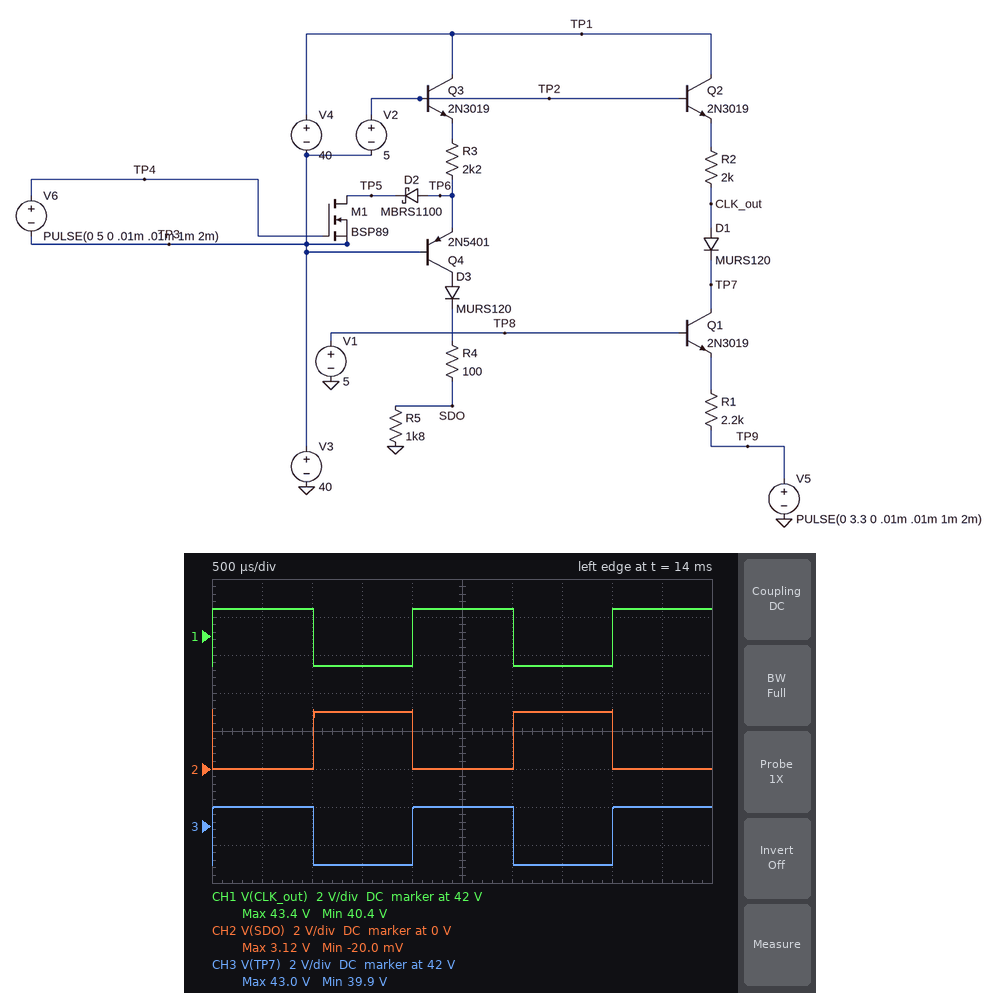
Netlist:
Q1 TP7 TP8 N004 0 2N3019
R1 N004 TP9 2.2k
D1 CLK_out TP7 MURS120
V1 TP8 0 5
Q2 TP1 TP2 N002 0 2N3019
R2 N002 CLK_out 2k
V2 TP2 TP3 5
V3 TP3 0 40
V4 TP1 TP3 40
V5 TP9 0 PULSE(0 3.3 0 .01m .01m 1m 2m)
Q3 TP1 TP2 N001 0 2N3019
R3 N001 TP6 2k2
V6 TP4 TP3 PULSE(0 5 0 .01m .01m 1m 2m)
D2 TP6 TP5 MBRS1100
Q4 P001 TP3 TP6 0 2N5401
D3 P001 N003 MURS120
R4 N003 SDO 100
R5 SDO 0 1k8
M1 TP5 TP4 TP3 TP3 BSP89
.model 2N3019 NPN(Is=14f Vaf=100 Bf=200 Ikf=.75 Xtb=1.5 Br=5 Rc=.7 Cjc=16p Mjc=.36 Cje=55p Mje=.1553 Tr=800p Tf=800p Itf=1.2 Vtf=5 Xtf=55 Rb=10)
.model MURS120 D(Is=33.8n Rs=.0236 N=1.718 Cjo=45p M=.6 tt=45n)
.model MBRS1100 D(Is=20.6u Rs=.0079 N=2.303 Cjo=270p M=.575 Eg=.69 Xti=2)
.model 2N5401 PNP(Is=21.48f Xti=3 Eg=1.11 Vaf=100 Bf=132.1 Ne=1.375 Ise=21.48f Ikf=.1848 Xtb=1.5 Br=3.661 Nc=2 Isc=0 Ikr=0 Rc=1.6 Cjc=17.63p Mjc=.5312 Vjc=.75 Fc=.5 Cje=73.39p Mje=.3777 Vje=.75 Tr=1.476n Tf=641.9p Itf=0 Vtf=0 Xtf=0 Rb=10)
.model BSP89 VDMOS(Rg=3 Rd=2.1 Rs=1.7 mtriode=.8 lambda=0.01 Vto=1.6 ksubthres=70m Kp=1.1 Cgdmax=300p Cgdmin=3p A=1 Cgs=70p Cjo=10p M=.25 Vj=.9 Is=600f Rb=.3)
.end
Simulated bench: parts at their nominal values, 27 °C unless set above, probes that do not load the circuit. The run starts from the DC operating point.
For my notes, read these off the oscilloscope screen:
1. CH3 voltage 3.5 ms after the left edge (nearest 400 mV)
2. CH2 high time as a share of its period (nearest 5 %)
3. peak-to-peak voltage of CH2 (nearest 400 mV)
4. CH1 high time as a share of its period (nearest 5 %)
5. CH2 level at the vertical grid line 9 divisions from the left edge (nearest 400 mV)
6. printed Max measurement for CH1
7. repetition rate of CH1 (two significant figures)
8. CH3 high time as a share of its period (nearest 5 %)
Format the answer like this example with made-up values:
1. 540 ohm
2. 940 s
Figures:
1. 40.0 V
2. 50 %
3. 3.2 V
4. 50 %
5. 0 V
6. 43.4 V
7. 500 Hz
8. 50 %
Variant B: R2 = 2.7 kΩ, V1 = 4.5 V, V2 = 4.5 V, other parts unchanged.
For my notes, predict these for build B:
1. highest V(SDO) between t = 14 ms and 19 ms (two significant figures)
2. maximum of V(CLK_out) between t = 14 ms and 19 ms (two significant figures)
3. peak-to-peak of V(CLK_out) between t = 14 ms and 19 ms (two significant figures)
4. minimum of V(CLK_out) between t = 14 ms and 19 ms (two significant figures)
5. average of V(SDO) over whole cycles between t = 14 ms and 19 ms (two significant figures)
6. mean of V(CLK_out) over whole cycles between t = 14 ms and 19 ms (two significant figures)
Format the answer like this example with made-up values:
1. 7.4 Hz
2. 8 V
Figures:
1. 2.7 V
2. 43 V
3. 4.0 V
4. 39 V
5. 1.3 V
6. 41 V
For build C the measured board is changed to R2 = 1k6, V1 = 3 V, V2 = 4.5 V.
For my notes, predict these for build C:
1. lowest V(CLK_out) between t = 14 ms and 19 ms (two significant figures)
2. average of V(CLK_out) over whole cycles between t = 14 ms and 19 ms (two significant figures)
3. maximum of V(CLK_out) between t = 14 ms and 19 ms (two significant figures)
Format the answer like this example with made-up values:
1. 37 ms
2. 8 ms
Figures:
1. 42 V
2. 43 V
3. 44 V
